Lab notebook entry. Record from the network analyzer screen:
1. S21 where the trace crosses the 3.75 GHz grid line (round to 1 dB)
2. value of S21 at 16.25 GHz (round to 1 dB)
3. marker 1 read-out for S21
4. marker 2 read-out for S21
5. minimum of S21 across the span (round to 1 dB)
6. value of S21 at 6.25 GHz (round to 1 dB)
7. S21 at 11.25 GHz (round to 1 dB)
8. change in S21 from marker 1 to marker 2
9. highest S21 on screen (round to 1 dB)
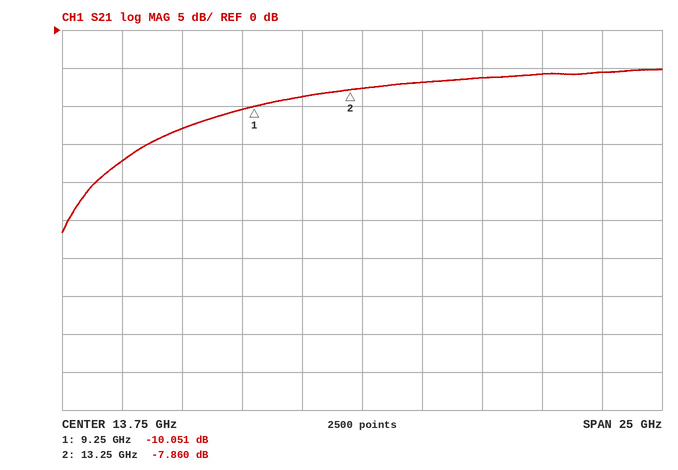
-17 dB
-7 dB
-10.051 dB
-7.860 dB
-27 dB
-13 dB
-9 dB
2.191 dB
-5 dB
